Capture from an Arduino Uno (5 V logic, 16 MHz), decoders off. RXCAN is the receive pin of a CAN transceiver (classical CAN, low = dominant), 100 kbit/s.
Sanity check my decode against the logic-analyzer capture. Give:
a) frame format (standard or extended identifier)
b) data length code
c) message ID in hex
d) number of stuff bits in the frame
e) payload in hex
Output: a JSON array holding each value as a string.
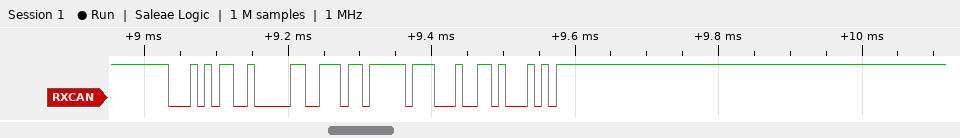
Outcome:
["standard", "2", "0x159", "2", "76 FF"]
